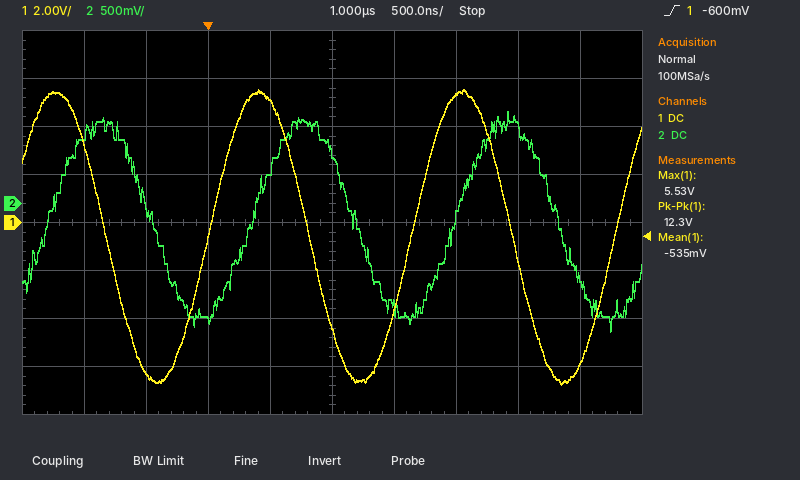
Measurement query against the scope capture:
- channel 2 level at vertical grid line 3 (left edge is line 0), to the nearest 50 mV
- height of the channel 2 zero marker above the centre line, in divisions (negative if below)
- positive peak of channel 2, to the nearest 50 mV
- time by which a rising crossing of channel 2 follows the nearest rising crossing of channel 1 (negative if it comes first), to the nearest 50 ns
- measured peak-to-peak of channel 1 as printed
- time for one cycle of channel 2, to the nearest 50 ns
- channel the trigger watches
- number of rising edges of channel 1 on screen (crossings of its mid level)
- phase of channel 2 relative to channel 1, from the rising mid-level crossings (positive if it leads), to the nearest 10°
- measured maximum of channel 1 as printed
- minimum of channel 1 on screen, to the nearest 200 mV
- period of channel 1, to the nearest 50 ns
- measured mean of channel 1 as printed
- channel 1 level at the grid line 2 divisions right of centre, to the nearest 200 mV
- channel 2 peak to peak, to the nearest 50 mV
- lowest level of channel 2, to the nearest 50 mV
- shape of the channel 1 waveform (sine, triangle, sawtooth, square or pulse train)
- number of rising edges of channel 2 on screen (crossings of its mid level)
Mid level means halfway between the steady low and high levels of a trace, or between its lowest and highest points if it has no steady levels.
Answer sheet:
-1.20 V
+0.4 div
950 mV
+350 ns
12.3 V
1.65 µs
channel 1
3
-80°
5.53 V
-6.8 V
1.65 µs
-535 mV
5.4 V
2.30 V
-1.35 V
sine
3
